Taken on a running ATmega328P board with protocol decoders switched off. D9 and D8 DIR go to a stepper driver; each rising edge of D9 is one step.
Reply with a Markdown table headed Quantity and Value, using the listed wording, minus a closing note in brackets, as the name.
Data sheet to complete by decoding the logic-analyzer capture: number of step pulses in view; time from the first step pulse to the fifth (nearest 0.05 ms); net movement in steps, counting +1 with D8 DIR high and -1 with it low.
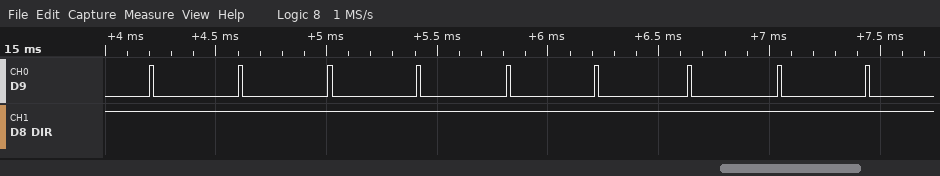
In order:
| Quantity | Value |
|---|---|
| number of step pulses in view | 9 |
| time from the first step pulse to the fifth | 1.60 ms |
| net movement in steps, counting +1 with D8 DIR high and -1 with it low | +9 |
